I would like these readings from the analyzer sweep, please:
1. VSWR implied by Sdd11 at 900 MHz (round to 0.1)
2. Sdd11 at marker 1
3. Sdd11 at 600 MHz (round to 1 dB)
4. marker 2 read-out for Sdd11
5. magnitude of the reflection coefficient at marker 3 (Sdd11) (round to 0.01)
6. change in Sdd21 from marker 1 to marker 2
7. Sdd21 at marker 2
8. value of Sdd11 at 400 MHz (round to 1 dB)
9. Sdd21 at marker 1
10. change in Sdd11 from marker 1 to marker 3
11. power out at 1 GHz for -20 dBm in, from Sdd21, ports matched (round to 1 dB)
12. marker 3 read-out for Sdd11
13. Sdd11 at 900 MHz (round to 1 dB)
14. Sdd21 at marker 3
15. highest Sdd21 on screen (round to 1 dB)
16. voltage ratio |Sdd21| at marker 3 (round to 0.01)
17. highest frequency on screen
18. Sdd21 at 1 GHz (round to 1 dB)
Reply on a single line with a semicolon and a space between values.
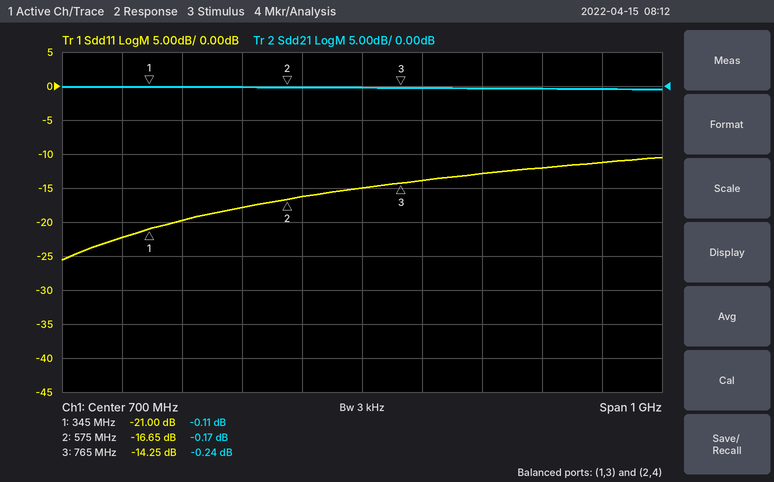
1.6; -21.00 dB; -16 dB; -16.65 dB; 0.19; -0.06 dB; -0.17 dB; -20 dB; -0.11 dB; 6.75 dB; -20 dBm; -14.25 dB; -13 dB; -0.24 dB; 0 dB; 0.97; 1.2 GHz; 0 dB
